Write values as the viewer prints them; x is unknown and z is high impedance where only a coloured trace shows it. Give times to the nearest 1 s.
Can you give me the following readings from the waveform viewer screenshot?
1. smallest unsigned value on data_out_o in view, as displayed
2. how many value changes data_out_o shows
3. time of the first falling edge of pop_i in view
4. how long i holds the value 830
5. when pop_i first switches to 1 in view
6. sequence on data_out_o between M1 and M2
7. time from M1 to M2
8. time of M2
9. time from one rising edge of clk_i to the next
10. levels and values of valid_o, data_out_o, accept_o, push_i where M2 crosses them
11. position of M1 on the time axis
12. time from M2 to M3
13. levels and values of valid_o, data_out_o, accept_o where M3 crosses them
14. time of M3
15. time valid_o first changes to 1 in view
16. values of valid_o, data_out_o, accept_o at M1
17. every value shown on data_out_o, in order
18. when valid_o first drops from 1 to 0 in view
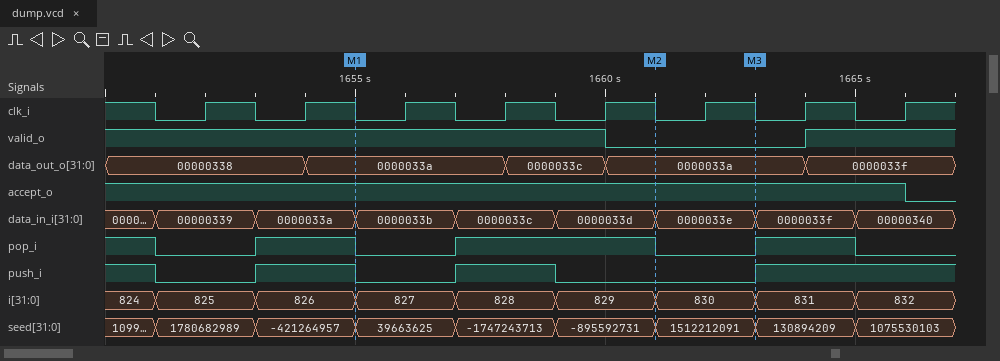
00000338
4
1651 s
2 s
1653 s
0000033a, 0000033c, 0000033a
6 s
1661 s
2 s
valid_o=0, data_out_o=0000033a, accept_o=1, push_i=0
1655 s
2 s
valid_o=0, data_out_o=0000033a, accept_o=1
1663 s
1664 s
valid_o=1, data_out_o=0000033a, accept_o=1
00000338, 0000033a, 0000033c, 0000033a, 0000033f
1660 s
